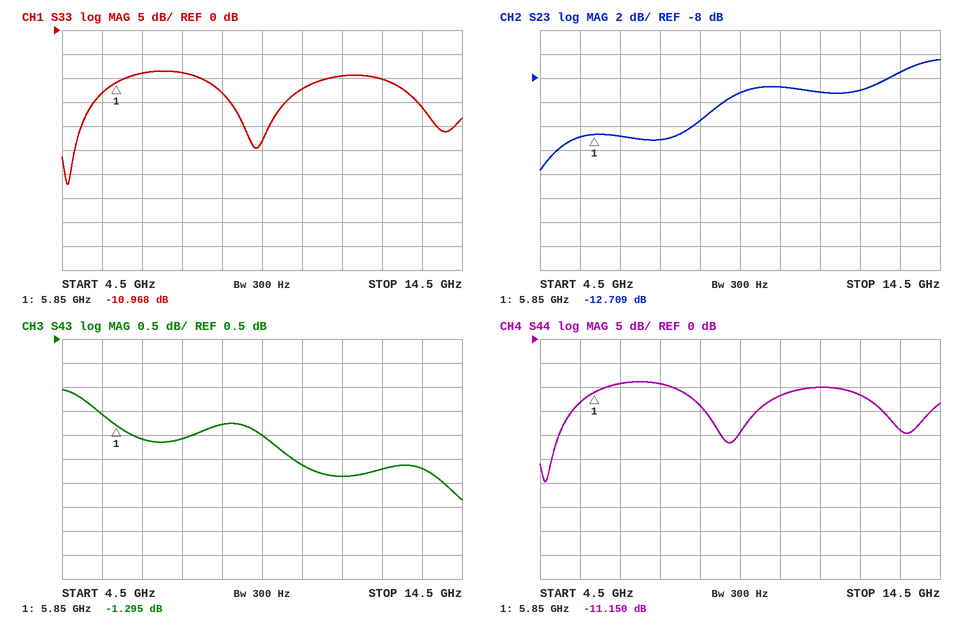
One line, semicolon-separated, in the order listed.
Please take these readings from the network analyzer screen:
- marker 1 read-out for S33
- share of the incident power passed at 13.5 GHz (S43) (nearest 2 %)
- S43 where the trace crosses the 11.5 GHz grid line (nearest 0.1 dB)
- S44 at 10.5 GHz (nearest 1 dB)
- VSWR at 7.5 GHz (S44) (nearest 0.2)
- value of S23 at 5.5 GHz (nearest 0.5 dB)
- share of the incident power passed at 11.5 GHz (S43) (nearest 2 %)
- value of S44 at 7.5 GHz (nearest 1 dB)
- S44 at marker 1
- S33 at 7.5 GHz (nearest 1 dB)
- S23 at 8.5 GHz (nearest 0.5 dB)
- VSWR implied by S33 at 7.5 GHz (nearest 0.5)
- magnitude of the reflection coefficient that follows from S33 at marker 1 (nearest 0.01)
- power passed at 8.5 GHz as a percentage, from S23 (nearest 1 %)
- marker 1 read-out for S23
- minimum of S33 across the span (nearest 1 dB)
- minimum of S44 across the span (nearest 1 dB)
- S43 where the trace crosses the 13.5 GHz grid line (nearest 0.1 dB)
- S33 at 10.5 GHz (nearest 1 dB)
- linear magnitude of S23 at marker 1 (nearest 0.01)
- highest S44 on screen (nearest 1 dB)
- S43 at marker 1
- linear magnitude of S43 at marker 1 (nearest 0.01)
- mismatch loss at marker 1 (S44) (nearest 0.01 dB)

-10.968 dB; 60 %; -2.4 dB; -12 dB; 2.0; -13.0 dB; 58 %; -9 dB; -11.150 dB; -9 dB; -11.5 dB; 2.0; 0.28; 7 %; -12.709 dB; -32 dB; -30 dB; -2.2 dB; -12 dB; 0.23; -9 dB; -1.295 dB; 0.86; 0.35 dB
